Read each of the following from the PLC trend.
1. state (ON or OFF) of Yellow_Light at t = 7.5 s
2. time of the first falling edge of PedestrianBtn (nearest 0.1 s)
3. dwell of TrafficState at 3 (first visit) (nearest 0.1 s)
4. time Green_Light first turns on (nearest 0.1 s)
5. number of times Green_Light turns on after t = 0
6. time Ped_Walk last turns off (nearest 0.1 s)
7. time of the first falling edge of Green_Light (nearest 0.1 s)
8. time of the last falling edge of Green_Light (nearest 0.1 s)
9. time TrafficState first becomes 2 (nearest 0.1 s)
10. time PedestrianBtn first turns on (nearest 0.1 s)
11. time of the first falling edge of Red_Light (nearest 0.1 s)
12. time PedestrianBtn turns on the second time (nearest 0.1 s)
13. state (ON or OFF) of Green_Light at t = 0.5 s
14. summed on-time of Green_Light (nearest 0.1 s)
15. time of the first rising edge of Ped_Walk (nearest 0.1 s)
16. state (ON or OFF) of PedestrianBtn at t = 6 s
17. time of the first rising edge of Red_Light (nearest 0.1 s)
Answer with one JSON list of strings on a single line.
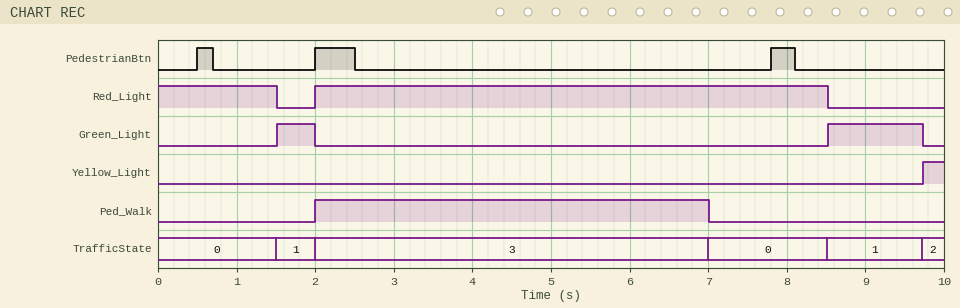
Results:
["OFF", "0.7 s", "5.0 s", "1.5 s", "2", "7.0 s", "2.0 s", "9.7 s", "9.7 s", "0.5 s", "1.5 s", "2.0 s", "OFF", "1.7 s", "2.0 s", "OFF", "2.0 s"]
